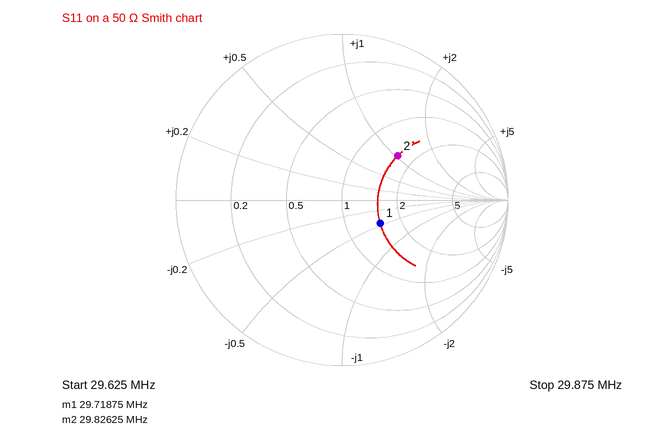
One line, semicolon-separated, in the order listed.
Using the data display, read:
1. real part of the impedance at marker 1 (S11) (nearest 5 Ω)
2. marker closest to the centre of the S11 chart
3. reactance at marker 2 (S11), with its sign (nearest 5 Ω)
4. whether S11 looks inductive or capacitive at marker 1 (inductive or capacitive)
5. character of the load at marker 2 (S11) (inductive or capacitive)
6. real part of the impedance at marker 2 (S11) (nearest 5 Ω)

75 Ω; marker 1; +50 Ω; capacitive; inductive; 80 Ω
